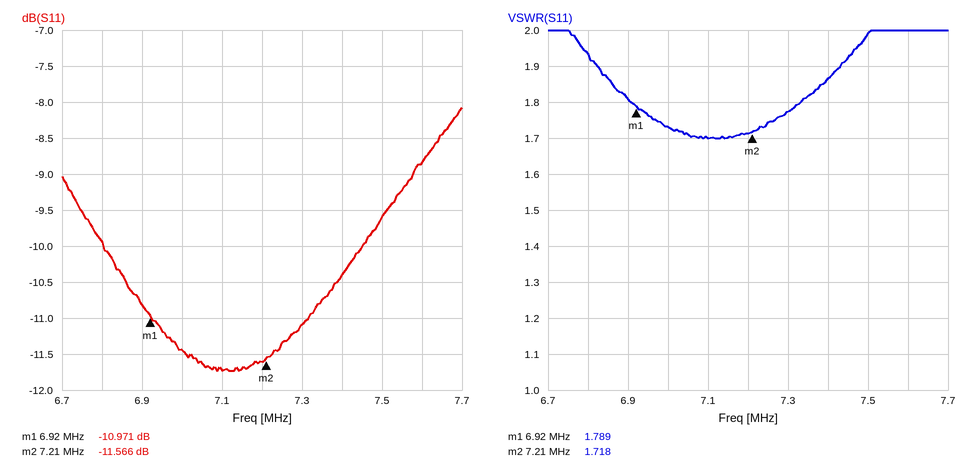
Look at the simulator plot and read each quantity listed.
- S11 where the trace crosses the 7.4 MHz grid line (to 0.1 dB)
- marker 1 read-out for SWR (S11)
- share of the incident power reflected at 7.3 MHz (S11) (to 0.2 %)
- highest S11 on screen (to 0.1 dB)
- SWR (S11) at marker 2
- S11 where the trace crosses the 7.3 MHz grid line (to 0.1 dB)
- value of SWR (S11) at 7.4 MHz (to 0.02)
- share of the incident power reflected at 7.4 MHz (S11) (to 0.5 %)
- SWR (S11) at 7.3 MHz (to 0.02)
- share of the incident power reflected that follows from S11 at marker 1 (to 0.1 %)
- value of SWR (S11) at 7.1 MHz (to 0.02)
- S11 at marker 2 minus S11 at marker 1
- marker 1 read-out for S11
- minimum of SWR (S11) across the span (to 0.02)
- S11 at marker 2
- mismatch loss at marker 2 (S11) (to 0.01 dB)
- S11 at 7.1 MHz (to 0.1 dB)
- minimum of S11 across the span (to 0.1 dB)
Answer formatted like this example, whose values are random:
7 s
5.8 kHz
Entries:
-10.4 dB
1.789
7.8 %
-8.1 dB
1.718
-11.1 dB
1.86
9.0 %
1.78
8.0 %
1.70
-0.595 dB
-10.971 dB
1.70
-11.566 dB
0.31 dB
-11.7 dB
-11.7 dB
